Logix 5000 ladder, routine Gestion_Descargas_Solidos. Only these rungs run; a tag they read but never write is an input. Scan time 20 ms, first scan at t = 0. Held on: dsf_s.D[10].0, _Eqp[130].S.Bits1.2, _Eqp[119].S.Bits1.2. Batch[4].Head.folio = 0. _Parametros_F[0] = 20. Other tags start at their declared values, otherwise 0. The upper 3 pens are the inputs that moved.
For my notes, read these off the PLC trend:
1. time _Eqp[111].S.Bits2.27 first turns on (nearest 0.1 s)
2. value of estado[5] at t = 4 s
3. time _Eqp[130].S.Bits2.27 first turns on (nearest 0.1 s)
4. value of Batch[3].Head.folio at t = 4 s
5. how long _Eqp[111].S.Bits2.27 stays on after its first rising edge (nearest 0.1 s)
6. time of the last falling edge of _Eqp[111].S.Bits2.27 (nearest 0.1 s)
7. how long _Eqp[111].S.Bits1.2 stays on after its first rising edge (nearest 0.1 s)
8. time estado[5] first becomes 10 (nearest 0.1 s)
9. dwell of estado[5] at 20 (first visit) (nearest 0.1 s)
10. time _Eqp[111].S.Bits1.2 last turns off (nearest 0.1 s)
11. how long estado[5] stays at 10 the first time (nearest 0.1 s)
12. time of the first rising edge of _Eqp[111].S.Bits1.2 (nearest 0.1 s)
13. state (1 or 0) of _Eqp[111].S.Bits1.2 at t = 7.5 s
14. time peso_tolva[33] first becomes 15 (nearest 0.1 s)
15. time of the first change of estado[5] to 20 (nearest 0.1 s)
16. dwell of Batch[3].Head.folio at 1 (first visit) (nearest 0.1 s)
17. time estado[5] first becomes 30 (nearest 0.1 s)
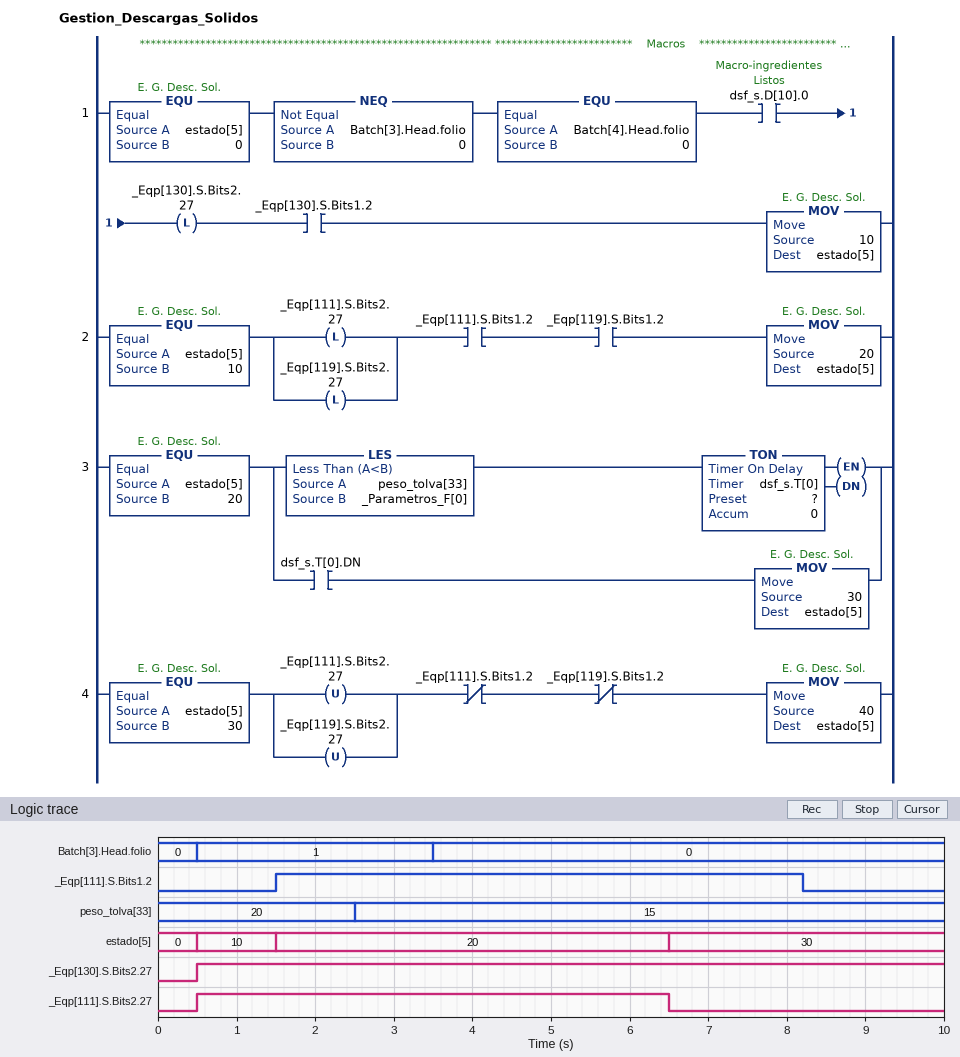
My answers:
0.5 s
20
0.5 s
0
6.0 s
6.5 s
6.7 s
0.5 s
5.0 s
8.2 s
1.0 s
1.5 s
1
2.5 s
1.5 s
3.0 s
6.5 s
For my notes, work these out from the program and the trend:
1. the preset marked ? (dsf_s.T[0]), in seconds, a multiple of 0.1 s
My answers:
4.0 s
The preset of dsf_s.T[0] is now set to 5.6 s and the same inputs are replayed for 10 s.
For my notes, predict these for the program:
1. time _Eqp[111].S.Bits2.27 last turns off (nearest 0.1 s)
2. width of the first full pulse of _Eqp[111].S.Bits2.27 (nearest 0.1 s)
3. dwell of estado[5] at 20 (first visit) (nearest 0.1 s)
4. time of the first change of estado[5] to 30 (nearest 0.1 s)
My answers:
8.1 s
7.6 s
6.6 s
8.1 s
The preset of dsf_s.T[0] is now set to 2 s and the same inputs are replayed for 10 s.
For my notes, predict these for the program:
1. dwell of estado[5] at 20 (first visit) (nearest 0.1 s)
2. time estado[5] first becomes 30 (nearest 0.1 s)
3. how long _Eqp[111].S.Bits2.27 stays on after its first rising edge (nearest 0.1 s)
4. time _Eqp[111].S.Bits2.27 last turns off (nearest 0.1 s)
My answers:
3.0 s
4.5 s
4.0 s
4.5 s
